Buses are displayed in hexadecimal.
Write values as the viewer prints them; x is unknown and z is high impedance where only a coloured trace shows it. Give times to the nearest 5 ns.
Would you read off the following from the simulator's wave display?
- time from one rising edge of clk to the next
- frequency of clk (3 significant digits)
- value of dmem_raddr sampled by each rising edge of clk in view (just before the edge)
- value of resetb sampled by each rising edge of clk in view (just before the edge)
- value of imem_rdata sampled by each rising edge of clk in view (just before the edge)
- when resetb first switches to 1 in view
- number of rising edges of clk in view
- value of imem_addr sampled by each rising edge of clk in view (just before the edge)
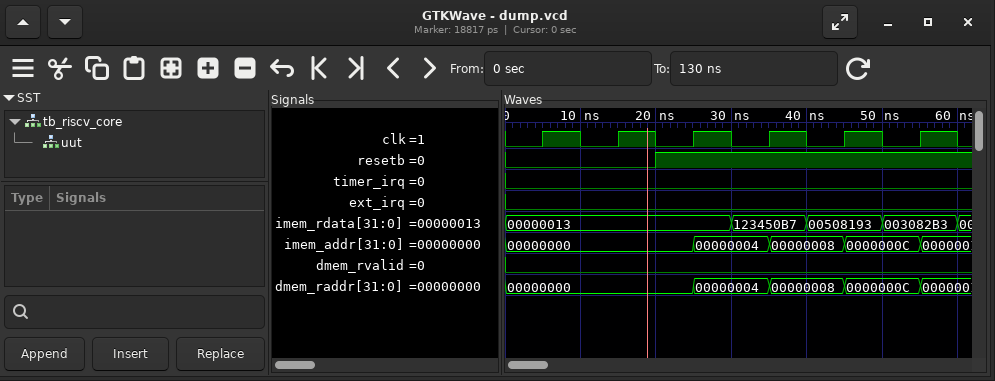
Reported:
10 ns
100 MHz
00000000, 00000000, 00000000, 00000004, 00000008, 0000000C
0 0 1 1 1 1
00000013, 00000013, 00000013, 123450B7, 00508193, 003082B3
20 ns
6
00000000, 00000000, 00000000, 00000004, 00000008, 0000000C
